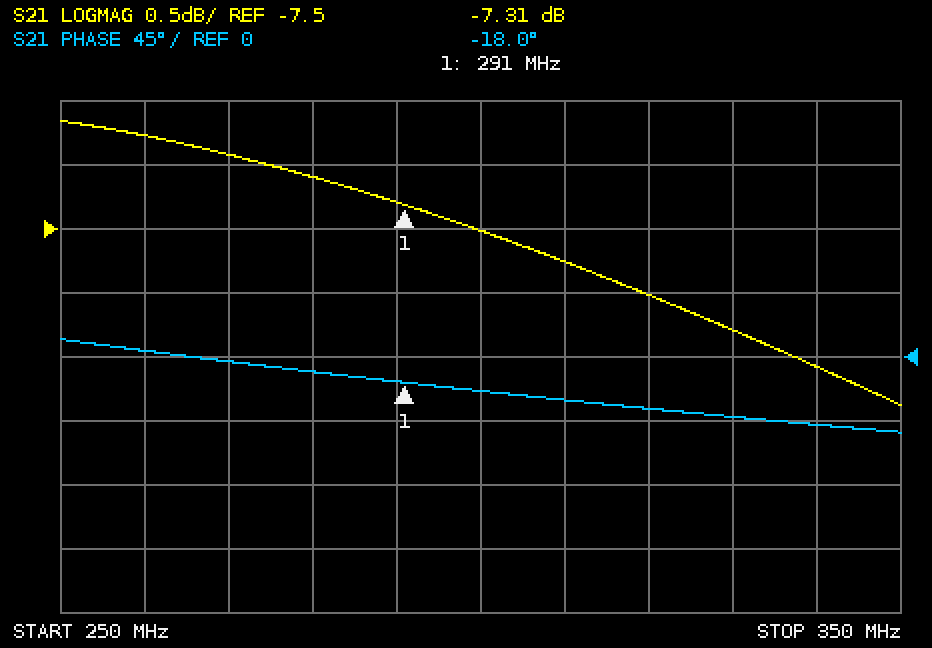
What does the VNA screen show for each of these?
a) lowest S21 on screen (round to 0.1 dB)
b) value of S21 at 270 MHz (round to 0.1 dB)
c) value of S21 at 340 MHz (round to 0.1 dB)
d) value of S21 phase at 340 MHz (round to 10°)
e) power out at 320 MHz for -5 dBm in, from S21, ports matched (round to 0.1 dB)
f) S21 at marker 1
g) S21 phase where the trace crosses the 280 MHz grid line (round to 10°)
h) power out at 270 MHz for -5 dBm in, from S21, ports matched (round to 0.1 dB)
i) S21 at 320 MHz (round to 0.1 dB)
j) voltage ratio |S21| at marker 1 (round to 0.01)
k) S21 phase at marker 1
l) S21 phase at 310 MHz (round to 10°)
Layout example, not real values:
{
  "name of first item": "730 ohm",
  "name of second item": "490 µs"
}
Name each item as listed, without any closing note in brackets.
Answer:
{
  "lowest S21 on screen": "-8.9 dB",
  "value of S21 at 270 MHz": "-6.9 dB",
  "value of S21 at 340 MHz": "-8.6 dB",
  "value of S21 phase at 340 MHz": "-50°",
  "power out at 320 MHz for -5 dBm in, from S21, ports matched": "-13.0 dBm",
  "S21 at marker 1": "-7.31 dB",
  "S21 phase where the trace crosses the 280 MHz grid line": "-10°",
  "power out at 270 MHz for -5 dBm in, from S21, ports matched": "-11.9 dBm",
  "S21 at 320 MHz": "-8.0 dB",
  "voltage ratio |S21| at marker 1": "0.43",
  "S21 phase at marker 1": "-18.0°",
  "S21 phase at 310 MHz": "-30°"
}
